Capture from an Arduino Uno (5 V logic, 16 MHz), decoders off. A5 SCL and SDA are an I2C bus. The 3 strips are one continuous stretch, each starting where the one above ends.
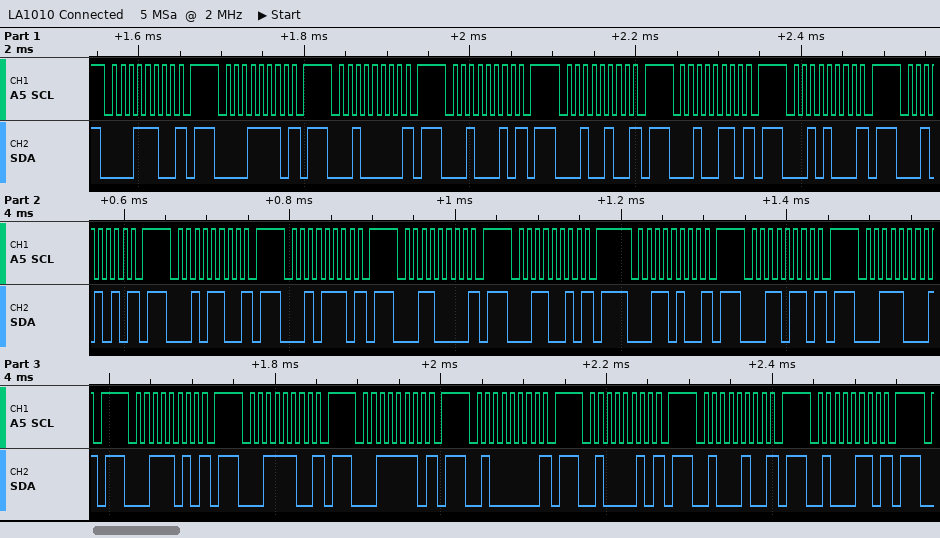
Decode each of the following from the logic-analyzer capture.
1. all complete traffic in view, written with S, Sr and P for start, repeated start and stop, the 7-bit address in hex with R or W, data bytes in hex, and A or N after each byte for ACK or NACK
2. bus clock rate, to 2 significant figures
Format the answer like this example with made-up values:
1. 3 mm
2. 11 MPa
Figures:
1. S 0EW N P S 0FW N P S 10W N P S 11W N P S 12W N P S 13W N P S 14W N P S 15W N P S 16W N P S 17W N P S 18W N P S 19W N P S 1AW N P S 1BW N P S 1CW N P S 1DW N P S 1EW N P S 1FW N P S 20W N P S 21W N P S 22W N P S 23W N P
2. 100 kHz
